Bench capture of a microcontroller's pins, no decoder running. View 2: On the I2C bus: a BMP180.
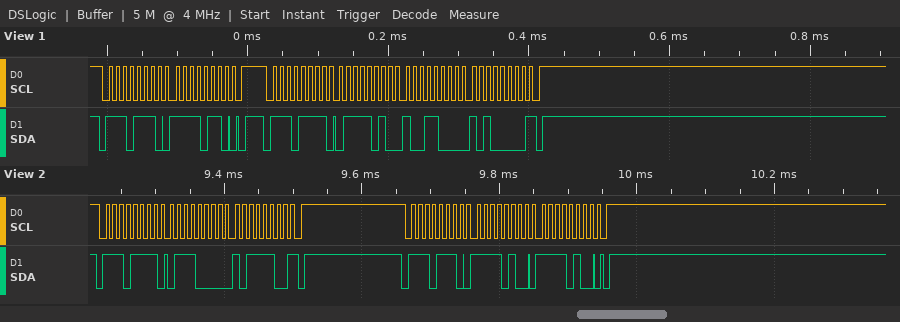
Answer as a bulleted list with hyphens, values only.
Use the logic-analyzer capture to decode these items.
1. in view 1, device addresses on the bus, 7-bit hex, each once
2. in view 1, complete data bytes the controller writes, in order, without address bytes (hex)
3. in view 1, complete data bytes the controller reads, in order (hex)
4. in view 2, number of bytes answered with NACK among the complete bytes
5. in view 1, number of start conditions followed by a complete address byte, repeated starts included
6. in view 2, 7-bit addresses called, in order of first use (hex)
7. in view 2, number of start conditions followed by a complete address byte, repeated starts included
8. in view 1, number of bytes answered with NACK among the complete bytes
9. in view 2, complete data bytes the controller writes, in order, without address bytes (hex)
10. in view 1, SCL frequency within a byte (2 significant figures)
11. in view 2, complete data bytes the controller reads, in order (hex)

- 0x77
- F6
- 7A 98 A0
- 1
- 2
- 0x77
- 2
- 1
- F4 F4
- 100 kHz
- 70 BC
